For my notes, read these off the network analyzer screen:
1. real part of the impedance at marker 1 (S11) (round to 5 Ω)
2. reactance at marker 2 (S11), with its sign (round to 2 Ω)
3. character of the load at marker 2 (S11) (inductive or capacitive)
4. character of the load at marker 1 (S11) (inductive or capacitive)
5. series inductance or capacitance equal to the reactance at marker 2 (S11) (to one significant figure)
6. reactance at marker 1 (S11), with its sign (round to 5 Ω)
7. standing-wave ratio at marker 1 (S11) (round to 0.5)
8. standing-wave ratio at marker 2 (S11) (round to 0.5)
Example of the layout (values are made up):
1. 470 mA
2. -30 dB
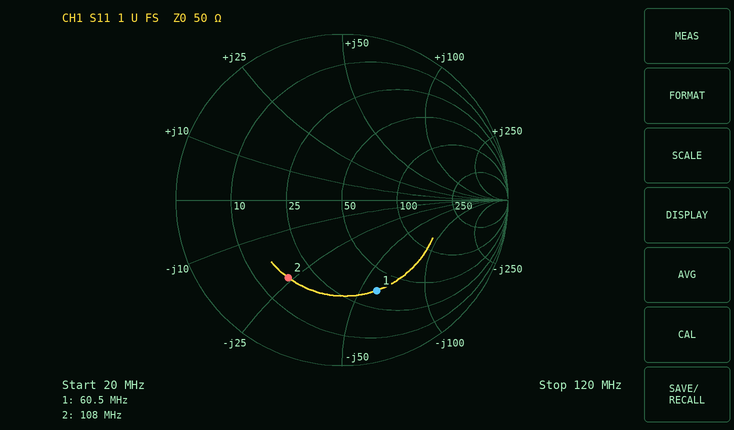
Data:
1. 35 Ω
2. -24 Ω
3. capacitive
4. capacitive
5. 60 pF
6. -60 Ω
7. 4.0
8. 3.5
